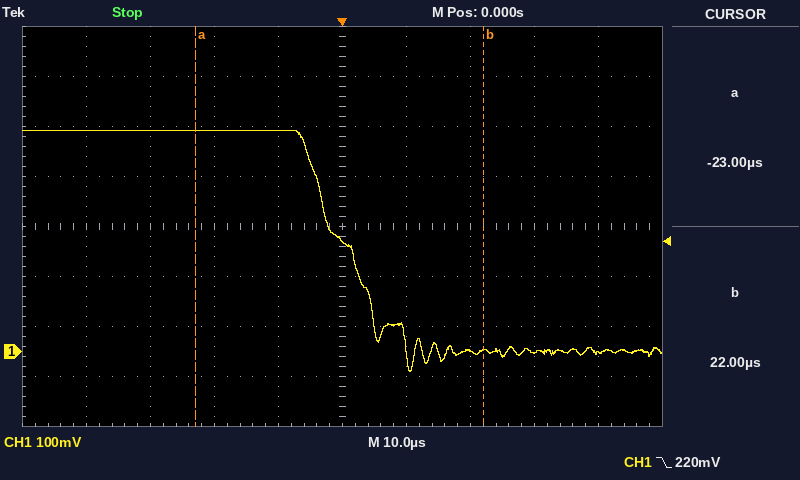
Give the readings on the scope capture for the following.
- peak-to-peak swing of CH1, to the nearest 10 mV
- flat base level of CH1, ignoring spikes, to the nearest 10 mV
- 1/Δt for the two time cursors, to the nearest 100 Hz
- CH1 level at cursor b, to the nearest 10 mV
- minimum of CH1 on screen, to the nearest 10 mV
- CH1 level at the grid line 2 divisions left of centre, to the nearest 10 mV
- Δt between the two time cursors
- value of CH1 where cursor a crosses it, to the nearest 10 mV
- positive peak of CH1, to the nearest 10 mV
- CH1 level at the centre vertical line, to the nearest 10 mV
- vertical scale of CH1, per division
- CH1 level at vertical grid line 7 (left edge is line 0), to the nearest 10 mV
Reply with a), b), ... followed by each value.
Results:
a) 480 mV
b) 0 mV
c) 22.2 kHz
d) 0 mV
e) -40 mV
f) 440 mV
g) 45 µs
h) 440 mV
i) 440 mV
j) 220 mV
k) 100 mV
l) 0 mV
